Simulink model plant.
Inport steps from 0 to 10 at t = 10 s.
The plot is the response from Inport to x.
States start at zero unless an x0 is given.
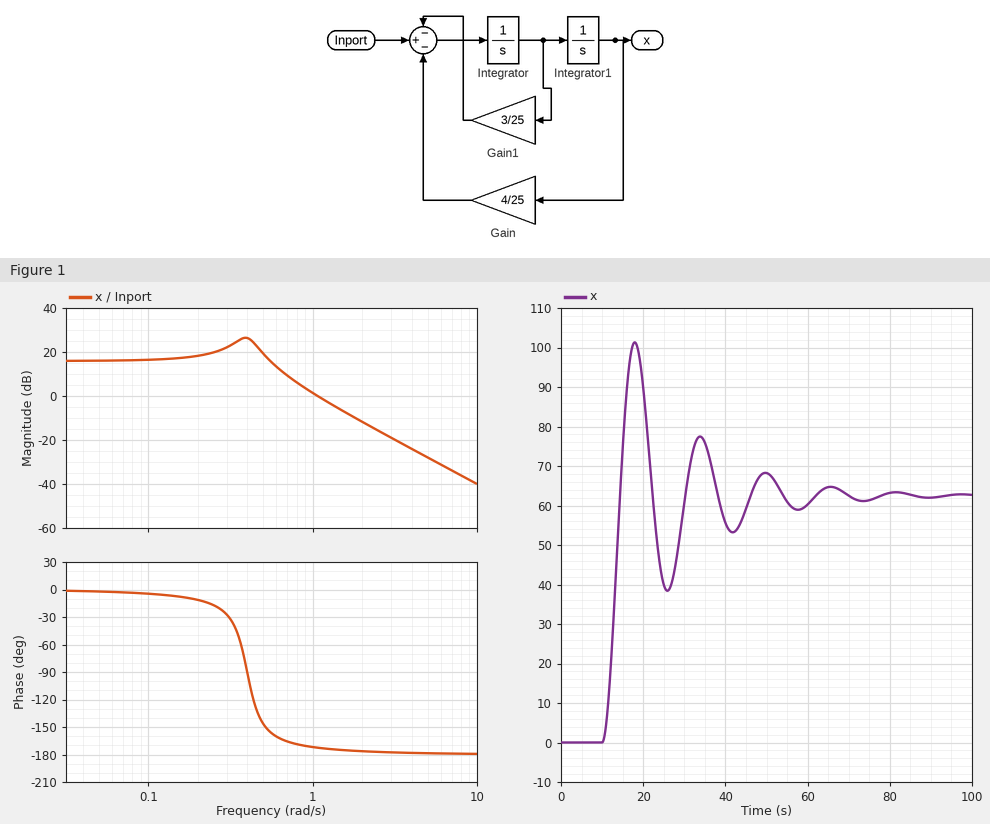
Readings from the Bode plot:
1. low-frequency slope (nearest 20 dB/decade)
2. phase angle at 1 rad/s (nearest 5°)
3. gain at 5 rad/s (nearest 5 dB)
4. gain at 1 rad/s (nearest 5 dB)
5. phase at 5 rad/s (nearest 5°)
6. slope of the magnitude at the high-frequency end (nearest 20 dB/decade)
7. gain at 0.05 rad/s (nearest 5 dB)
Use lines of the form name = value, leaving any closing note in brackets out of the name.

low-frequency slope = 0 dB/decade
phase angle at 1 rad/s = -170°
gain at 5 rad/s = -30 dB
gain at 1 rad/s = 0 dB
phase at 5 rad/s = -180°
slope of the magnitude at the high-frequency end = -40 dB/decade
gain at 0.05 rad/s = 15 dB
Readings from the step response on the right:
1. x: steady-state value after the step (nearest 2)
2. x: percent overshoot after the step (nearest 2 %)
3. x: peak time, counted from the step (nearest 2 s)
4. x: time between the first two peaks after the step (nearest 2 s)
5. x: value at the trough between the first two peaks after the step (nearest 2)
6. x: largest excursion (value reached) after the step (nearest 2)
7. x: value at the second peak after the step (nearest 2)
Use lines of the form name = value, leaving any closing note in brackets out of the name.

x: steady-state value after the step = 62
x: percent overshoot after the step = 62 %
x: peak time, counted from the step = 8 s
x: time between the first two peaks after the step = 16 s
x: value at the trough between the first two peaks after the step = 38
x: largest excursion (value reached) after the step = 102
x: value at the second peak after the step = 78
